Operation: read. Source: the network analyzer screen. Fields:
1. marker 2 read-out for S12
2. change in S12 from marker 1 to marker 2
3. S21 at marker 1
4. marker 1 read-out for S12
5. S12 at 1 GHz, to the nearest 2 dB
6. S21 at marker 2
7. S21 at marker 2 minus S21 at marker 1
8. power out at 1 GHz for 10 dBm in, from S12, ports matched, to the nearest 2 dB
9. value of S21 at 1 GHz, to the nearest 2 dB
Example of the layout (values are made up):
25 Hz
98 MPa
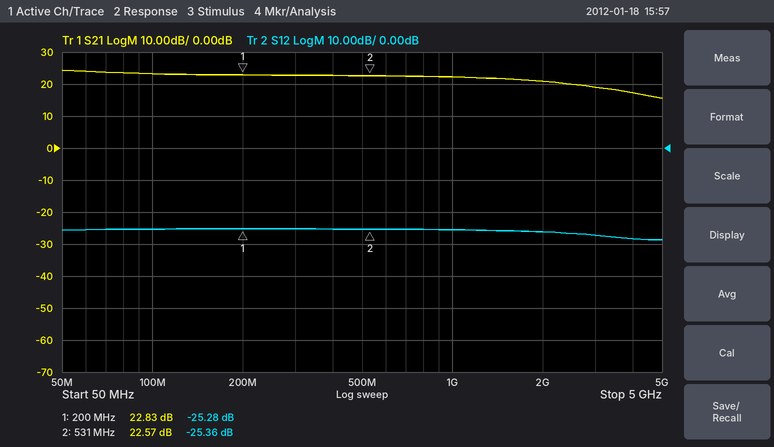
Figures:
-25.36 dB
-0.08 dB
22.83 dB
-25.28 dB
-26 dB
22.57 dB
-0.26 dB
-16 dBm
22 dB
